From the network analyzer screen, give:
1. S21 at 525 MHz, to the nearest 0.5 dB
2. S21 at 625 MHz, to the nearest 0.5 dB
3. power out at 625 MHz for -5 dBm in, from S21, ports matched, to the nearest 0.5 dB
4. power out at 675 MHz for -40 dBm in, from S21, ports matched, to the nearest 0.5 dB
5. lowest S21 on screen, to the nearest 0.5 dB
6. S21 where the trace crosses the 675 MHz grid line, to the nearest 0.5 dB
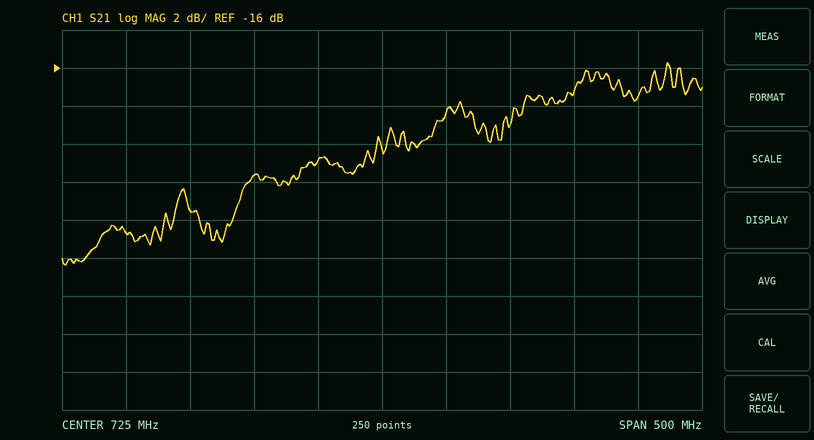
-24.5 dB
-21.5 dB
-26.5 dBm
-61.0 dBm
-26.5 dB
-21.0 dB
